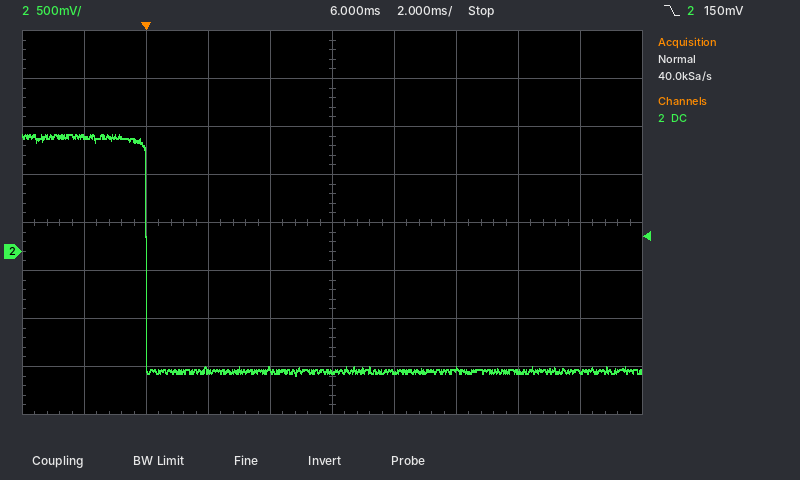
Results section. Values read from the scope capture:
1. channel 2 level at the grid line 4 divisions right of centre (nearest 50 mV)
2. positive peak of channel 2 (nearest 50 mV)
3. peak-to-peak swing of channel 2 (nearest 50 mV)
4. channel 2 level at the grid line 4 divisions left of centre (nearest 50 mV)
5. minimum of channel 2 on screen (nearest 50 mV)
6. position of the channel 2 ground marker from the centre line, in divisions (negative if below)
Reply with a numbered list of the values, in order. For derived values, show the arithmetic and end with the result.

1. -1.25 V
2. 1.20 V
3. 1.20 V − (-1.30 V) = 2.50 V
4. 1.20 V
5. -1.30 V
6. -0.6 div
